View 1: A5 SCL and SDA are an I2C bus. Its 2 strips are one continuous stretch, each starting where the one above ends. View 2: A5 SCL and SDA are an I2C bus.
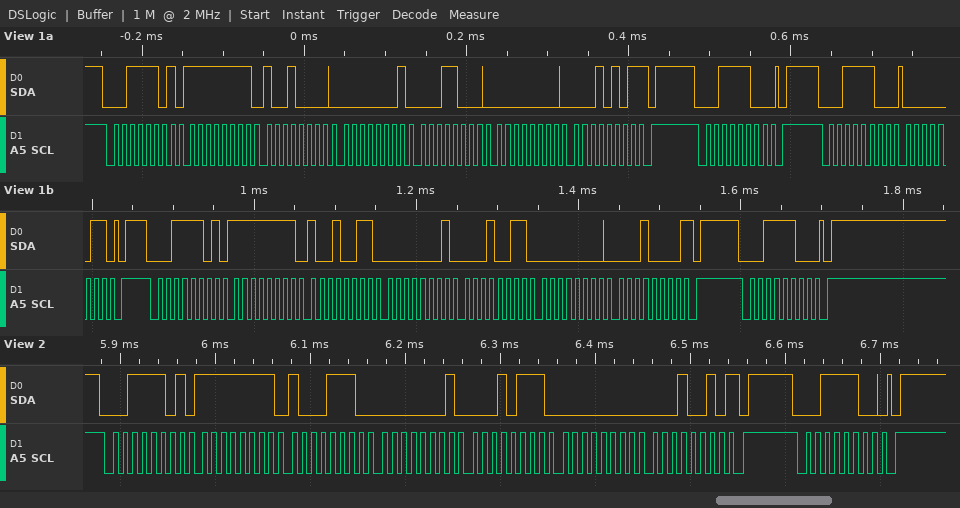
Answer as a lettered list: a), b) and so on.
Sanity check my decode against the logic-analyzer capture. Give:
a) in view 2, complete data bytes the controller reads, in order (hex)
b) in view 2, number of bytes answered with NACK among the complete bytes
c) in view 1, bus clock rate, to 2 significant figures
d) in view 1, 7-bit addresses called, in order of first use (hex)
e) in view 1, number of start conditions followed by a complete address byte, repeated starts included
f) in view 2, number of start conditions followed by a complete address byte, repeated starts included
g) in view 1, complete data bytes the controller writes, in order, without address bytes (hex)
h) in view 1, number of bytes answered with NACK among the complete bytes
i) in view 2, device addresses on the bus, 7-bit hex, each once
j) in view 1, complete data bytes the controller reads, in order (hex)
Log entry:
a) FF 8E 01 17 00 12
b) 1
c) 100 kHz
d) 0x1E
e) 5
f) 2
g) 03
h) 2
i) 0x1E
j) FF 90 01 18 00 15 FF 93 01 13 00 10
